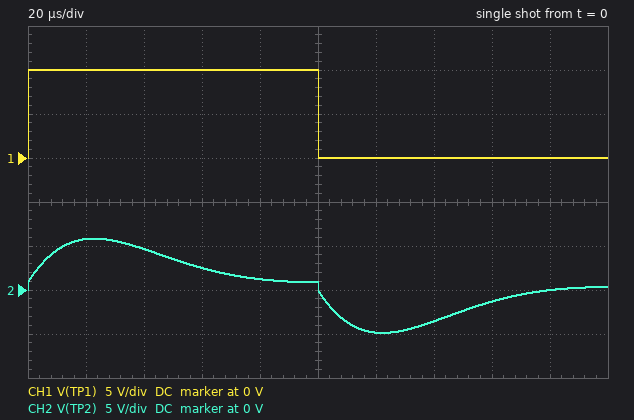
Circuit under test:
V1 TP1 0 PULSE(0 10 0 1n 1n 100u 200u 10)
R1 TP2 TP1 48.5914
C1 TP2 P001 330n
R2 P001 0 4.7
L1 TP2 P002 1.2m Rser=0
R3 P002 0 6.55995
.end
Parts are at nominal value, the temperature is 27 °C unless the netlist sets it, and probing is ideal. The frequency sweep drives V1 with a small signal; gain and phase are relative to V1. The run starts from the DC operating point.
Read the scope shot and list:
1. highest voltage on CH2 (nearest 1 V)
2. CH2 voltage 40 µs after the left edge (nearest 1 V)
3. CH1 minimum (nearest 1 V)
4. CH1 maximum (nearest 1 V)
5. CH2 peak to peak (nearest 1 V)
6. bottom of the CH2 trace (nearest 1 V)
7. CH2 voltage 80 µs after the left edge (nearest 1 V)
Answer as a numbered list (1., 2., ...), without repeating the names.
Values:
1. 6 V
2. 5 V
3. 0 V
4. 10 V
5. 11 V
6. -5 V
7. 1 V
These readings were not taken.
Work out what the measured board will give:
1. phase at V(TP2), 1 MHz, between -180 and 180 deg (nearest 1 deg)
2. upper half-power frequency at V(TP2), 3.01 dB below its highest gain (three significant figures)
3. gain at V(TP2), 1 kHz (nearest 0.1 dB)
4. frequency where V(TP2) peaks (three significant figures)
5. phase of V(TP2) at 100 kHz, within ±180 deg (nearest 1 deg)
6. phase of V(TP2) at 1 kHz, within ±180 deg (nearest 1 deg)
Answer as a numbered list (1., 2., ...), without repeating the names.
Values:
1. -5 deg
2. 15.0 kHz
3. -14.8 dB
4. 8.12 kHz
5. -40 deg
6. 40 deg
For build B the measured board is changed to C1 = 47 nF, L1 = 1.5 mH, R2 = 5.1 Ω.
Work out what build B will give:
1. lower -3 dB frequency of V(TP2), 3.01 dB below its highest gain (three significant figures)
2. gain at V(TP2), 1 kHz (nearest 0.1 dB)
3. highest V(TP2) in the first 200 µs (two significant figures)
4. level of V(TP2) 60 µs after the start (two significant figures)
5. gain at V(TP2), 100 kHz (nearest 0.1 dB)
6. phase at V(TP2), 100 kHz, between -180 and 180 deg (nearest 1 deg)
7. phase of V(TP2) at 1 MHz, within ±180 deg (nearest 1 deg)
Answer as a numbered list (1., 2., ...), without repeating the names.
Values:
1. 5.24 kHz
2. -13.7 dB
3. 8.5 V
4. 2.2 V
5. -5.2 dB
6. -48 deg
7. -30 deg
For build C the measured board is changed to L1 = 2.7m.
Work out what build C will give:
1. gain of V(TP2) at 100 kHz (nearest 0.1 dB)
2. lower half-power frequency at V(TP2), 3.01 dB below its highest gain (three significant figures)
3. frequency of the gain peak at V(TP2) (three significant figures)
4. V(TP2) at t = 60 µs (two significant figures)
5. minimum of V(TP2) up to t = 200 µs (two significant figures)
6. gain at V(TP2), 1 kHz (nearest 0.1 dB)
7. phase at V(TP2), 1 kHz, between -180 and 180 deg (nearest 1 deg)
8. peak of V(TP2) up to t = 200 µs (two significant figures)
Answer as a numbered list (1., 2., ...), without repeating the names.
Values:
1. -18.0 dB
2. 2.40 kHz
3. 5.41 kHz
4. 5.4 V
5. -5.3 V
6. -9.8 dB
7. 51 deg
8. 7.0 V
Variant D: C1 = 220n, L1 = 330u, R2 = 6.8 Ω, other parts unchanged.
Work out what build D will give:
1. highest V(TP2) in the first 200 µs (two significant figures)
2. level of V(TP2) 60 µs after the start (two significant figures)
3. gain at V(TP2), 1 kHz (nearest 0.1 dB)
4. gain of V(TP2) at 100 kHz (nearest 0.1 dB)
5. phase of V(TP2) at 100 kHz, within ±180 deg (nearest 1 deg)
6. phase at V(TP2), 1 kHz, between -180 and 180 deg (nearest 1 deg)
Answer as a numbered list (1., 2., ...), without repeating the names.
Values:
1. 4.4 V
2. 1.1 V
3. -18.1 dB
4. -14.8 dB
5. -37 deg
6. 15 deg
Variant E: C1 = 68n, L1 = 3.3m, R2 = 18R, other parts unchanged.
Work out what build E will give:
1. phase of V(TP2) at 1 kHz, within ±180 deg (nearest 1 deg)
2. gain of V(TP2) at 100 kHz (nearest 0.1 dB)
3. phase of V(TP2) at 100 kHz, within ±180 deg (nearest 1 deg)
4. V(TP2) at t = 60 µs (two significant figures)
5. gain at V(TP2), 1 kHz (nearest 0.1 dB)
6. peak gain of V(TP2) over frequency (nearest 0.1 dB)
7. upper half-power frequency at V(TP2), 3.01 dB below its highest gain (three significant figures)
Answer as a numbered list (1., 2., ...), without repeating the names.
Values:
1. 52 deg
2. -7.5 dB
3. -33 deg
4. 4.7 V
5. -8.6 dB
6. -0.2 dB
7. 41.6 kHz
